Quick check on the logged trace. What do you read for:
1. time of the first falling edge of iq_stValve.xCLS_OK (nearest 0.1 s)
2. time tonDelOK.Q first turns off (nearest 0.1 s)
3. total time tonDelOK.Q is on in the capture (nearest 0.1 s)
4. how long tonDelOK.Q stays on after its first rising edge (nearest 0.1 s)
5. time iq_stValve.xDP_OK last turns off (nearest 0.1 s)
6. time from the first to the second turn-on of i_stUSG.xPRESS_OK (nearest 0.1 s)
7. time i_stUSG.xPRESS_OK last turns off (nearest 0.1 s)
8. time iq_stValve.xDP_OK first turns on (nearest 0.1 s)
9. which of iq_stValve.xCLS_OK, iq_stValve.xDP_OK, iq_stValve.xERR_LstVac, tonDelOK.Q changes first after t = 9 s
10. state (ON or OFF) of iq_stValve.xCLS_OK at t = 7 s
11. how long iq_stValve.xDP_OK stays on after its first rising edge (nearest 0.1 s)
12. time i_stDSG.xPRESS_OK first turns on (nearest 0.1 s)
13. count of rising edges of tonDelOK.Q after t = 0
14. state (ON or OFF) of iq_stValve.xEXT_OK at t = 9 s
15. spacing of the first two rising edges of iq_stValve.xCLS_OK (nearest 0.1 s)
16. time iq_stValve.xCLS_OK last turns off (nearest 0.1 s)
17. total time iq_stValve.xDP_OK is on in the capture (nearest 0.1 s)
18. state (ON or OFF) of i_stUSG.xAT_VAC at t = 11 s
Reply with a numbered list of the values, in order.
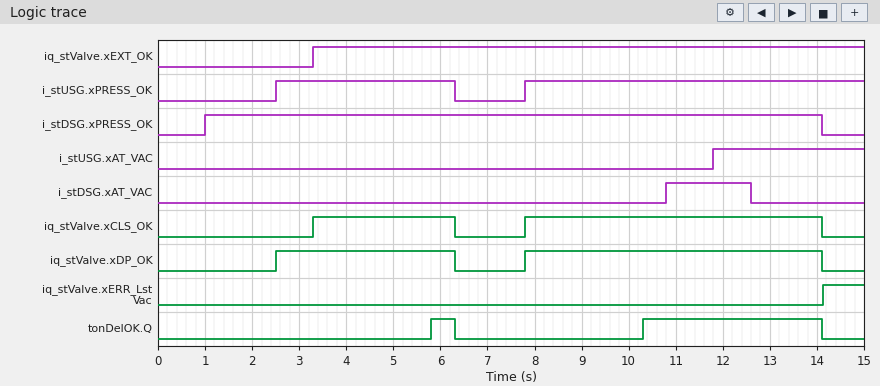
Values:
1. 6.3 s
2. 6.3 s
3. 4.3 s
4. 0.5 s
5. 14.1 s
6. 5.3 s
7. 6.3 s
8. 2.5 s
9. tonDelOK.Q
10. OFF
11. 3.8 s
12. 1.0 s
13. 2
14. ON
15. 4.5 s
16. 14.1 s
17. 10.1 s
18. OFF
